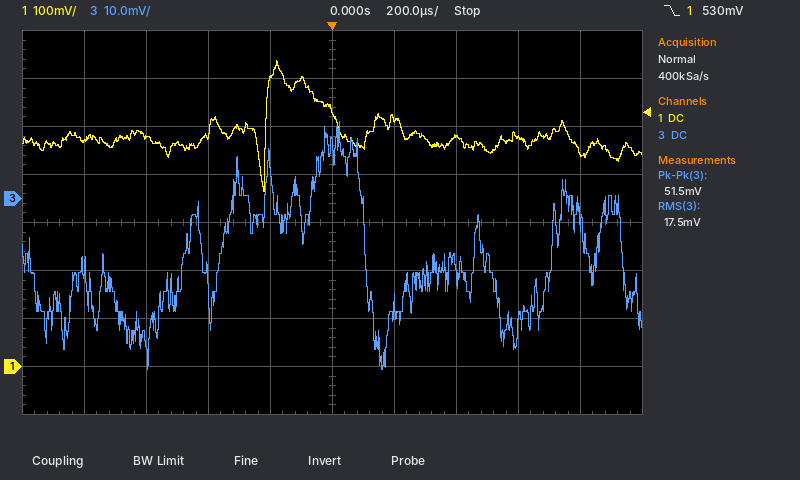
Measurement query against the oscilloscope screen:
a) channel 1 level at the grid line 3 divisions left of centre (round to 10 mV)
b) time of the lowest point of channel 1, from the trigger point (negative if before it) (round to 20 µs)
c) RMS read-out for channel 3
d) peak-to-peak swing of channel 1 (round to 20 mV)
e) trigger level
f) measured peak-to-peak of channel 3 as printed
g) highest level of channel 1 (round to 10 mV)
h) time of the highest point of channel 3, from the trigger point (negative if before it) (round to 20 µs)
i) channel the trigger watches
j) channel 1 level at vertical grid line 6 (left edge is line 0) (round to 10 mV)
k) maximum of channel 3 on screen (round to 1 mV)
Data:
480 mV
-220 µs
17.5 mV
280 mV
530 mV
51.5 mV
640 mV
+20 µs
channel 1
520 mV
16 mV
